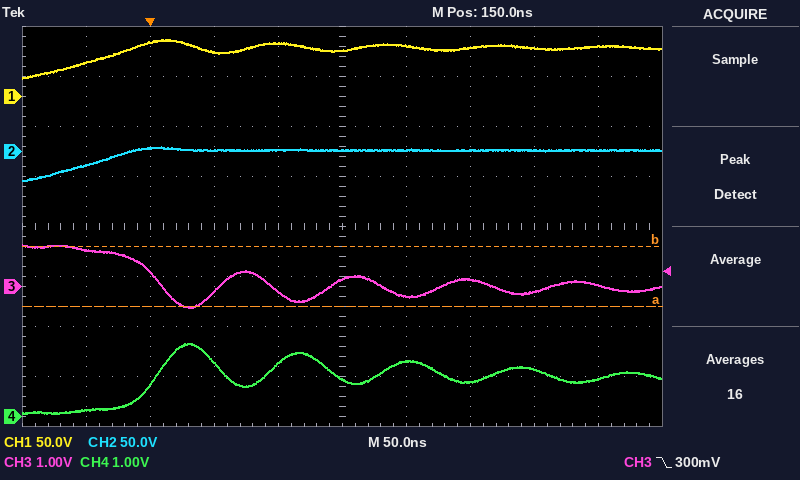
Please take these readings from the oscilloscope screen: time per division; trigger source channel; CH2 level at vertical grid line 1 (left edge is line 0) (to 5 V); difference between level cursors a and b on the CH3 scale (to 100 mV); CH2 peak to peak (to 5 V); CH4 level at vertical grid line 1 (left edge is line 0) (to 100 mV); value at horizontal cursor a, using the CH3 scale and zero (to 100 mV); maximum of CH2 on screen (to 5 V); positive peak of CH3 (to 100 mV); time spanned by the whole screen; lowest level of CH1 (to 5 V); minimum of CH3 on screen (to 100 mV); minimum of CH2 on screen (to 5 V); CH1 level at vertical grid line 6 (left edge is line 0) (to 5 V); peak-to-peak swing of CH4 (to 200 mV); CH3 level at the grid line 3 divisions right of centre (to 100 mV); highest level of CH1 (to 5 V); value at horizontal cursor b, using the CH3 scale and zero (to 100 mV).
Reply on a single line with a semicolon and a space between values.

50 ns; CH3; -15 V; 1.2 V; 35 V; 100 mV; -400 mV; 5 V; 800 mV; 500 ns; 20 V; -400 mV; -30 V; 50 V; 1.4 V; -100 mV; 55 V; 800 mV
